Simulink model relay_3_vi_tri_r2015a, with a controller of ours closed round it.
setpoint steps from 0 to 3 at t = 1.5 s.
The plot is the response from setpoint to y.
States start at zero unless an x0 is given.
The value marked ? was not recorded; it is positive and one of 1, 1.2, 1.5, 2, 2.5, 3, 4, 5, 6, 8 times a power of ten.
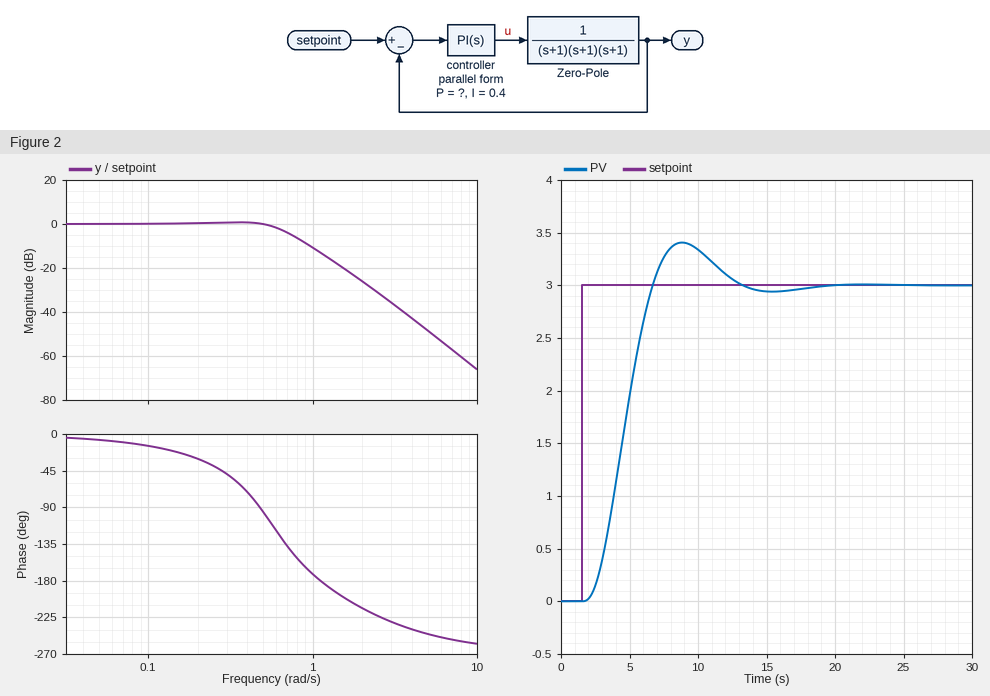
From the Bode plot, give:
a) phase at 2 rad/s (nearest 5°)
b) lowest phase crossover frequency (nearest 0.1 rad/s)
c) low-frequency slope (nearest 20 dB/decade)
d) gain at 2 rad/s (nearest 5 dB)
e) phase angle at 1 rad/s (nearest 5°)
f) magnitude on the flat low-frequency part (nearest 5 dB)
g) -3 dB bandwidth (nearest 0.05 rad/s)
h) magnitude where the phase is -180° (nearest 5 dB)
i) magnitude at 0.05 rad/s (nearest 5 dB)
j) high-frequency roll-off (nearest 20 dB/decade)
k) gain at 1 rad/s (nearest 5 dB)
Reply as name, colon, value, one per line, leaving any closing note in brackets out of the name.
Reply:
phase at 2 rad/s: -215°
lowest phase crossover frequency: 1.1 rad/s
low-frequency slope: 0 dB/decade
gain at 2 rad/s: -25 dB
phase angle at 1 rad/s: -170°
magnitude on the flat low-frequency part: 0 dB
-3 dB bandwidth: 0.65 rad/s
magnitude where the phase is -180°: -15 dB
magnitude at 0.05 rad/s: 0 dB
high-frequency roll-off: -60 dB/decade
gain at 1 rad/s: -10 dB
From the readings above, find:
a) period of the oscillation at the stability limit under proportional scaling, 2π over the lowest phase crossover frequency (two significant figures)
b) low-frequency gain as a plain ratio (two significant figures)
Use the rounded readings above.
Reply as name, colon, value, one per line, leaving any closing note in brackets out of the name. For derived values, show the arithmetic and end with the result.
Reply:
period of the oscillation at the stability limit under proportional scaling, 2π over the lowest phase crossover frequency: 2π / 1.1 = 5.7 s
low-frequency gain as a plain ratio: 10^(0 / 20) = 1.0
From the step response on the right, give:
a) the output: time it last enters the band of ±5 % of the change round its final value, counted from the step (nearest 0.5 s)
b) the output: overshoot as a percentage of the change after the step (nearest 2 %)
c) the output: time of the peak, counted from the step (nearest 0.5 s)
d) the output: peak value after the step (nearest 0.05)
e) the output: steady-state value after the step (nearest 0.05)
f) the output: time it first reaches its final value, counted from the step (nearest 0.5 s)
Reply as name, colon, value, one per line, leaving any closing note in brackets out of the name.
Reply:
the output: time it last enters the band of ±5 % of the change round its final value, counted from the step: 10.0 s
the output: overshoot as a percentage of the change after the step: 14 %
the output: time of the peak, counted from the step: 7.5 s
the output: peak value after the step: 3.40
the output: steady-state value after the step: 3.00
the output: time it first reaches its final value, counted from the step: 5.0 s
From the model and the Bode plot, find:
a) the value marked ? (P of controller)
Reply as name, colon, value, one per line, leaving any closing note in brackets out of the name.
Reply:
the value marked ?: 0.5
